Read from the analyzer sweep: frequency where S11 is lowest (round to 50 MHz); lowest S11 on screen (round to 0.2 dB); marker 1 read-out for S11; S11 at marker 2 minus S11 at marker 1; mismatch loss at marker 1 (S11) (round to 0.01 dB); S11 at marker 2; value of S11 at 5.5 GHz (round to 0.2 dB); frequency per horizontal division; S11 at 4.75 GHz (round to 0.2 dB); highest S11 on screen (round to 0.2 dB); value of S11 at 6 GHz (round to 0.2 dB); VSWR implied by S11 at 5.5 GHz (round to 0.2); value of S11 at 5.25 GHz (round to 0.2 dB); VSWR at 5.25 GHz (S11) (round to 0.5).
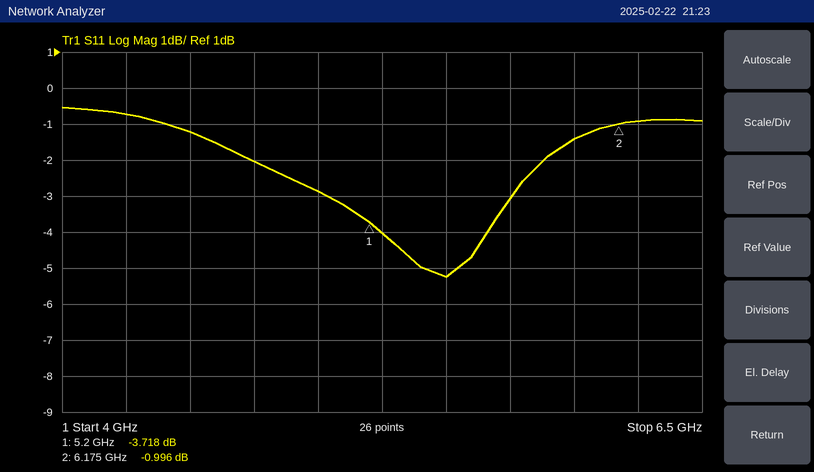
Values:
5.50 GHz
-5.2 dB
-3.718 dB
2.722 dB
2.40 dB
-0.996 dB
-5.2 dB
250 MHz
-2.0 dB
-0.6 dB
-1.4 dB
3.4
-4.0 dB
4.5
